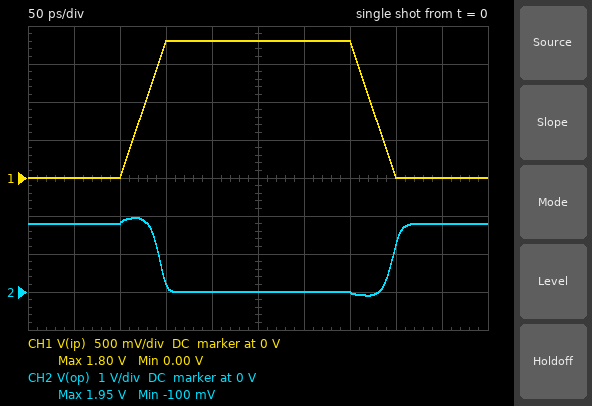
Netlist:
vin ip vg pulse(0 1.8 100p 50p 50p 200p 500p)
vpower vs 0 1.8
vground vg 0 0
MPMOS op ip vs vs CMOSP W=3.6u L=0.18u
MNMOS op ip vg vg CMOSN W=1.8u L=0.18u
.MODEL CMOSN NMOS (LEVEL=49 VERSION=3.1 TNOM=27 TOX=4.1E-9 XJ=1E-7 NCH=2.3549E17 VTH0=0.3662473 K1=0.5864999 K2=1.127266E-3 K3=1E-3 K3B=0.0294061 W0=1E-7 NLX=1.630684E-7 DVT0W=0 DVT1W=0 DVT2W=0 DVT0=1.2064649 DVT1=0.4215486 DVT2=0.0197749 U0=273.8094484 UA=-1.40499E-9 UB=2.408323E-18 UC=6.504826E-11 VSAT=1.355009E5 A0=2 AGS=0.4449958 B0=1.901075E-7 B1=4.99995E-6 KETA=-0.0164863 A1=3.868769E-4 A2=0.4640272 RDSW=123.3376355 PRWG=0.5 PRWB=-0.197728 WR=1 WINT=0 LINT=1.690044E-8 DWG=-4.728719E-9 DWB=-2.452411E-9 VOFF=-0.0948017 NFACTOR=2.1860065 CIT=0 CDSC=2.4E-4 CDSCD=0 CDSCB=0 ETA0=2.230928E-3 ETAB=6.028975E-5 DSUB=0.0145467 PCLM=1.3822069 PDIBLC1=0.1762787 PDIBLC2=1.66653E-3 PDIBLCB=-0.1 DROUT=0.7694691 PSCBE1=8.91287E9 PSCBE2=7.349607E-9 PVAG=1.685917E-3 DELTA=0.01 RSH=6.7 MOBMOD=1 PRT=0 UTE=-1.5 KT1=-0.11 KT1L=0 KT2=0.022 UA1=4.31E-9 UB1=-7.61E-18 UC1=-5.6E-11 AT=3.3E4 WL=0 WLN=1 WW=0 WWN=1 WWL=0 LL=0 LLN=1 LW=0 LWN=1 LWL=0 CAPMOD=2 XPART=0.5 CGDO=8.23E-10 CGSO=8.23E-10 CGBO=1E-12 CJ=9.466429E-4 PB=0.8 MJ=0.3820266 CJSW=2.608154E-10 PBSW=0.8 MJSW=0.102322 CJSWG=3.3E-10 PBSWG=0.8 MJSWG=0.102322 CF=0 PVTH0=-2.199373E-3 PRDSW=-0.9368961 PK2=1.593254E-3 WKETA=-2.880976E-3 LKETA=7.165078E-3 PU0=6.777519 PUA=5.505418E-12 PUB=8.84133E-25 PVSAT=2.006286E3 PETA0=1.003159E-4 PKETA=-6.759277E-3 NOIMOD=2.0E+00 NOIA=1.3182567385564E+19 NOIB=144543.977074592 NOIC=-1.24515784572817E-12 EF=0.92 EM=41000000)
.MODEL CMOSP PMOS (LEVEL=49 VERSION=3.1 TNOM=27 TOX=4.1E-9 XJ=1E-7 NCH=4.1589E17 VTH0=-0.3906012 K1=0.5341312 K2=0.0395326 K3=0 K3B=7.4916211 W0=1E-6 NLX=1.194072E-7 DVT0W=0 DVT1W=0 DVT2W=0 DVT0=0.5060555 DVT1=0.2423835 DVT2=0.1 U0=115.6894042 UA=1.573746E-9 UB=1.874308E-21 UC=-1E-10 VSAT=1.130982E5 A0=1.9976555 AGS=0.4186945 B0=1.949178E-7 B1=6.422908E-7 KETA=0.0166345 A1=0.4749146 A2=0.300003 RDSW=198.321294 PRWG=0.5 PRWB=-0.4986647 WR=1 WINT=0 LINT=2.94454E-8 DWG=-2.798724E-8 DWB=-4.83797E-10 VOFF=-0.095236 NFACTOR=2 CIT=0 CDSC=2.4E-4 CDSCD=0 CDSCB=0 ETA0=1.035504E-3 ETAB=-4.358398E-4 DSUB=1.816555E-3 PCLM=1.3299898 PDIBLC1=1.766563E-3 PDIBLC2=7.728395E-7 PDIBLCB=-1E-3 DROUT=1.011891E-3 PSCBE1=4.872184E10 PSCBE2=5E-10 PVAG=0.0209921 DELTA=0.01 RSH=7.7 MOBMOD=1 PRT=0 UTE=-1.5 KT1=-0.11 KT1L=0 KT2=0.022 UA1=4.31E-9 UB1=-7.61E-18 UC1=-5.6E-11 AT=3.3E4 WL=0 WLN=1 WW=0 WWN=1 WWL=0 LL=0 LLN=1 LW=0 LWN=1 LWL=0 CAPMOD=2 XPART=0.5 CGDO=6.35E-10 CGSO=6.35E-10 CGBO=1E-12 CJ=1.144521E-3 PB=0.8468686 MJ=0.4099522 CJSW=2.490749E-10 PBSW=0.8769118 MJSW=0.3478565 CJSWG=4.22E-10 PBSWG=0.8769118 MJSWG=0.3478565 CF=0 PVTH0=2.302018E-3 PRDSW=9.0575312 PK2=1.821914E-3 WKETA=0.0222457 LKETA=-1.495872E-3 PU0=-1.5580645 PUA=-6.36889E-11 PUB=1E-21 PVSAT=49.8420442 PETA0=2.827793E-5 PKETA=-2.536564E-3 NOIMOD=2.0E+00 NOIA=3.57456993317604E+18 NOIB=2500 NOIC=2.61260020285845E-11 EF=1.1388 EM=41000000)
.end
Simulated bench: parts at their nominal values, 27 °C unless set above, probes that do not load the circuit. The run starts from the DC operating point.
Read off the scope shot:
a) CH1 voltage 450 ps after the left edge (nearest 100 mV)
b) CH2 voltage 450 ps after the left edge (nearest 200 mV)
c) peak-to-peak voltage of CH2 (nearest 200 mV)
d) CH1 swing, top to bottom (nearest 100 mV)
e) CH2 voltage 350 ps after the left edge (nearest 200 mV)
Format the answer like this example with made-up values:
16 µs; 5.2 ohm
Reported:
0 V; 1.8 V; 2.0 V; 1.8 V; 0 V
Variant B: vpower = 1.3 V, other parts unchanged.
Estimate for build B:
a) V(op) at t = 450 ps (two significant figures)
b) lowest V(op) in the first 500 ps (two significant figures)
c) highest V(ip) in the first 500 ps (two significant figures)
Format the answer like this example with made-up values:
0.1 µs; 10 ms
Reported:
1.3 V; -210 mV; 1.8 V
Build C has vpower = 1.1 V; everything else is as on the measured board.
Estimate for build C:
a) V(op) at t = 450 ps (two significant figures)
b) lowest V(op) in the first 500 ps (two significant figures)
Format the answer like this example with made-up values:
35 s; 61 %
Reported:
1.1 V; -320 mV
